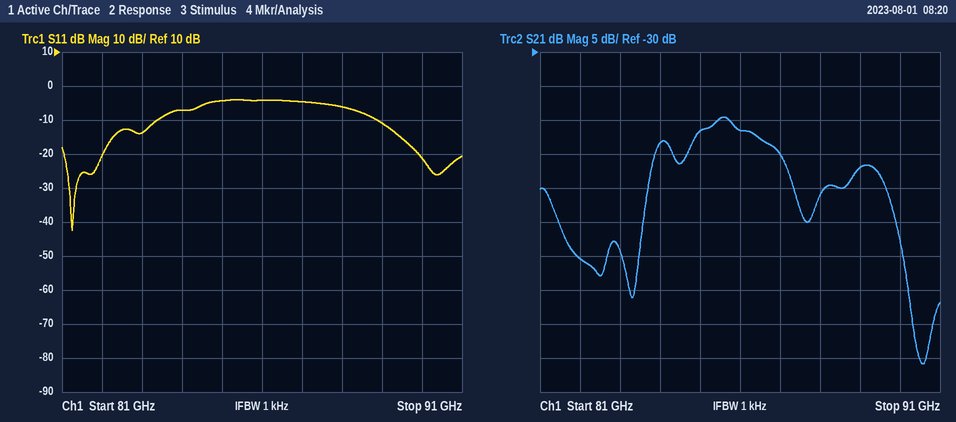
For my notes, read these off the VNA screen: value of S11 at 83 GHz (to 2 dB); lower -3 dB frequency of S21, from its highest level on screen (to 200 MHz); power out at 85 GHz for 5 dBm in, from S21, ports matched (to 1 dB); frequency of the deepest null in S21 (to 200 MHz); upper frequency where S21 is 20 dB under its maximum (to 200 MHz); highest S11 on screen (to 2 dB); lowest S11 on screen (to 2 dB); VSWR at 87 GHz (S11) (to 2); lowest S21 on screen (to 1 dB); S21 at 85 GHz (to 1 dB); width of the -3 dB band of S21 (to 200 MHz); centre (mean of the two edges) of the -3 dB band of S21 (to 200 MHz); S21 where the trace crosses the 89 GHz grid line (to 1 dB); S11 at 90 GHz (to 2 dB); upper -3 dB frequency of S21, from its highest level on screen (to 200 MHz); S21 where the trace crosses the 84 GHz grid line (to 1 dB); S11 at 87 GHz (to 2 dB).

-14 dB
84.8 GHz
-37 dBm
90.6 GHz
90.0 GHz
-4 dB
-42 dB
4
-76 dB
-42 dB
1.6 GHz
85.6 GHz
-47 dB
-22 dB
86.4 GHz
-43 dB
-4 dB
